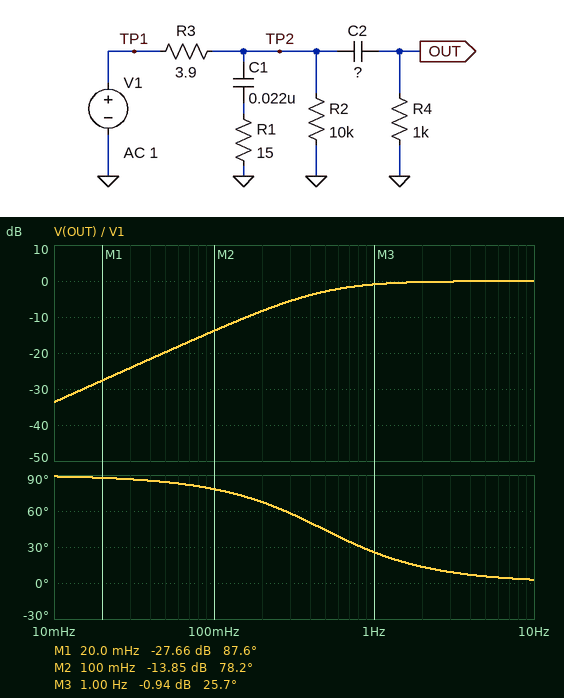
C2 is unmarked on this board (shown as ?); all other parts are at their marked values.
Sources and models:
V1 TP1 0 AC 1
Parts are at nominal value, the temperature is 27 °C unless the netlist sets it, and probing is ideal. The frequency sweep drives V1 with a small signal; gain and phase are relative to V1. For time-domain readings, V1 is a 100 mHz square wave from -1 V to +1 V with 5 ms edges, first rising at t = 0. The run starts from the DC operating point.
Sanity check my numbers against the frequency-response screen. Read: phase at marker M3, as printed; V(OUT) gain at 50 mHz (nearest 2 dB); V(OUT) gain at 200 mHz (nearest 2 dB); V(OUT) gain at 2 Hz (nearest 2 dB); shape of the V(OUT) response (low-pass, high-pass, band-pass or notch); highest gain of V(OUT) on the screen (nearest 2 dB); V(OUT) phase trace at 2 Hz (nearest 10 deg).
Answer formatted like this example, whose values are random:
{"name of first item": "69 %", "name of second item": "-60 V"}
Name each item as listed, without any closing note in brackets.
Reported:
{"phase at marker M3, as printed": "25.7 deg", "V(OUT) gain at 50 mHz": "-20 dB", "V(OUT) gain at 200 mHz": "-8 dB", "V(OUT) gain at 2 Hz": "0 dB", "shape of the V(OUT) response": "high-pass", "highest gain of V(OUT) on the screen": "0 dB", "V(OUT) phase trace at 2 Hz": "10 deg"}
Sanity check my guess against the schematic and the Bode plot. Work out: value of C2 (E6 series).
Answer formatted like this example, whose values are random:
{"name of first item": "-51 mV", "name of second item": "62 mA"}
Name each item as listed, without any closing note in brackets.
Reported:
{"value of C2": "330 µF"}
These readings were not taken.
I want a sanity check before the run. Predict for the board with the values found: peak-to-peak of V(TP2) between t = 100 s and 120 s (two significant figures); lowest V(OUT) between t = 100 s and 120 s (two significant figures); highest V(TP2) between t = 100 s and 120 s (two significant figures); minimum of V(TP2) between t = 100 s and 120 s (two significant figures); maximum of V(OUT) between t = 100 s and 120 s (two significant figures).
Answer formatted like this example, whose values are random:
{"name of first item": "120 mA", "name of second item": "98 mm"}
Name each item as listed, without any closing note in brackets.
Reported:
{"peak-to-peak of V(TP2) between t = 100 s and 120 s": "2.0 V", "lowest V(OUT) between t = 100 s and 120 s": "-2.0 V", "highest V(TP2) between t = 100 s and 120 s": "1.0 V", "minimum of V(TP2) between t = 100 s and 120 s": "-1.0 V", "maximum of V(OUT) between t = 100 s and 120 s": "2.0 V"}
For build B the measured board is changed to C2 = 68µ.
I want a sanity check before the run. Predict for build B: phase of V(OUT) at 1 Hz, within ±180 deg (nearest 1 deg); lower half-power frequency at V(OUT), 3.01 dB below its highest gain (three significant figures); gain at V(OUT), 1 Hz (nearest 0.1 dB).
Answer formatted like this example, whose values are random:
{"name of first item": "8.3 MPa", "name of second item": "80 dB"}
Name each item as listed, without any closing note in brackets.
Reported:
{"phase of V(OUT) at 1 Hz, within ±180 deg": "67 deg", "lower half-power frequency at V(OUT), 3.01 dB below its highest gain": "2.33 Hz", "gain at V(OUT), 1 Hz": "-8.1 dB"}
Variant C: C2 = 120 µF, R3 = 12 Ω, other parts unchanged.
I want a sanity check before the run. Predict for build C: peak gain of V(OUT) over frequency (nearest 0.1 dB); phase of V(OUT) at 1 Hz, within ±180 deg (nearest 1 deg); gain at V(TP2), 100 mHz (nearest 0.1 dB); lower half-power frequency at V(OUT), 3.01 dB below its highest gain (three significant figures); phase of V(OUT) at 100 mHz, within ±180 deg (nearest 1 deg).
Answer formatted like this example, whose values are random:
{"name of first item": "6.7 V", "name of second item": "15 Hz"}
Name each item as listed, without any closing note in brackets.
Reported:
{"peak gain of V(OUT) over frequency": "-0.1 dB", "phase of V(OUT) at 1 Hz, within ±180 deg": "53 deg", "gain at V(TP2), 100 mHz": "0 dB", "lower half-power frequency at V(OUT), 3.01 dB below its highest gain": "1.31 Hz", "phase of V(OUT) at 100 mHz, within ±180 deg": "86 deg"}
